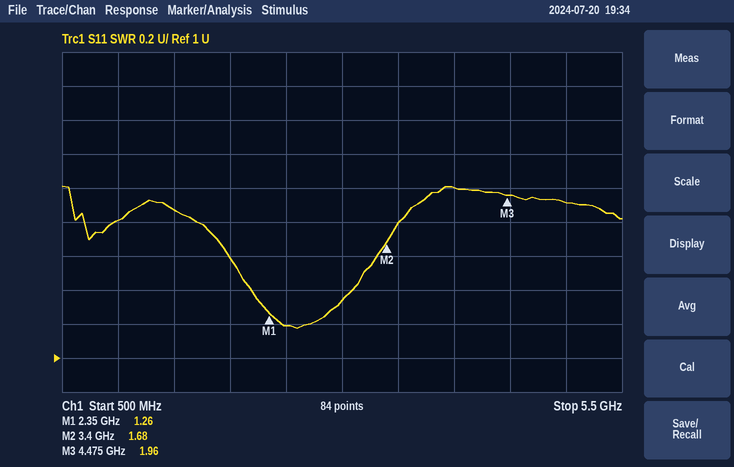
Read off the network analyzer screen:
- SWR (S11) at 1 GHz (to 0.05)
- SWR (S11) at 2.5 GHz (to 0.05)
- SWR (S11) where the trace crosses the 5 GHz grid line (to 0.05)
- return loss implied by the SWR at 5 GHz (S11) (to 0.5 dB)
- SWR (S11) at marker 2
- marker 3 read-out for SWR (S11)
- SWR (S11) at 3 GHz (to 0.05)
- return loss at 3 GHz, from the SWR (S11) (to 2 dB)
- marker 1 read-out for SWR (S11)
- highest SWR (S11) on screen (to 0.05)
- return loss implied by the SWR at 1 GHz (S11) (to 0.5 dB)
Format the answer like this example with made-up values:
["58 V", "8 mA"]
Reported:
["1.80", "1.20", "1.90", "10.0 dB", "1.68", "1.96", "1.35", "16 dB", "1.26", "2.00", "11.0 dB"]
